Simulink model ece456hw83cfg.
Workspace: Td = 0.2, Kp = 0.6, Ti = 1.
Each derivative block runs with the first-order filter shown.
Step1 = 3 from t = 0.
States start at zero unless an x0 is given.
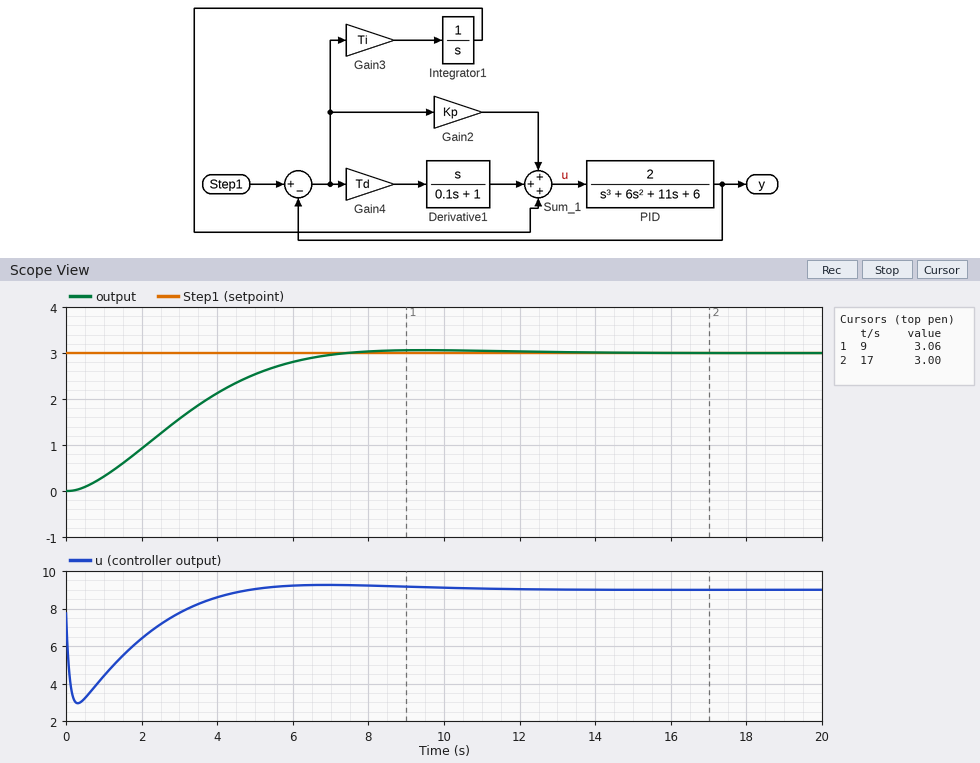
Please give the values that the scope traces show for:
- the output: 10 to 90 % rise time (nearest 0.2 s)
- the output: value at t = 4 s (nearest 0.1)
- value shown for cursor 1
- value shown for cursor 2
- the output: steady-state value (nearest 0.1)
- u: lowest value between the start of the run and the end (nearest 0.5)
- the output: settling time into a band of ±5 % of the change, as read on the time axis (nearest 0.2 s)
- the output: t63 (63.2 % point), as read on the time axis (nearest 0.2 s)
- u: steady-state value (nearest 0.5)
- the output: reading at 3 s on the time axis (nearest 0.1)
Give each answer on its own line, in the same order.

4.6 s
2.1
3.06
3.00
3.0
3.0
6.2 s
3.6 s
9.0
1.6
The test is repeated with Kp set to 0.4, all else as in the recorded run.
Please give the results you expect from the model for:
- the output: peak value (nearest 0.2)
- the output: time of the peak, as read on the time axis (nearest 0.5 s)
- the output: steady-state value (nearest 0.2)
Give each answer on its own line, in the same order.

3.2
9.0 s
3.0
